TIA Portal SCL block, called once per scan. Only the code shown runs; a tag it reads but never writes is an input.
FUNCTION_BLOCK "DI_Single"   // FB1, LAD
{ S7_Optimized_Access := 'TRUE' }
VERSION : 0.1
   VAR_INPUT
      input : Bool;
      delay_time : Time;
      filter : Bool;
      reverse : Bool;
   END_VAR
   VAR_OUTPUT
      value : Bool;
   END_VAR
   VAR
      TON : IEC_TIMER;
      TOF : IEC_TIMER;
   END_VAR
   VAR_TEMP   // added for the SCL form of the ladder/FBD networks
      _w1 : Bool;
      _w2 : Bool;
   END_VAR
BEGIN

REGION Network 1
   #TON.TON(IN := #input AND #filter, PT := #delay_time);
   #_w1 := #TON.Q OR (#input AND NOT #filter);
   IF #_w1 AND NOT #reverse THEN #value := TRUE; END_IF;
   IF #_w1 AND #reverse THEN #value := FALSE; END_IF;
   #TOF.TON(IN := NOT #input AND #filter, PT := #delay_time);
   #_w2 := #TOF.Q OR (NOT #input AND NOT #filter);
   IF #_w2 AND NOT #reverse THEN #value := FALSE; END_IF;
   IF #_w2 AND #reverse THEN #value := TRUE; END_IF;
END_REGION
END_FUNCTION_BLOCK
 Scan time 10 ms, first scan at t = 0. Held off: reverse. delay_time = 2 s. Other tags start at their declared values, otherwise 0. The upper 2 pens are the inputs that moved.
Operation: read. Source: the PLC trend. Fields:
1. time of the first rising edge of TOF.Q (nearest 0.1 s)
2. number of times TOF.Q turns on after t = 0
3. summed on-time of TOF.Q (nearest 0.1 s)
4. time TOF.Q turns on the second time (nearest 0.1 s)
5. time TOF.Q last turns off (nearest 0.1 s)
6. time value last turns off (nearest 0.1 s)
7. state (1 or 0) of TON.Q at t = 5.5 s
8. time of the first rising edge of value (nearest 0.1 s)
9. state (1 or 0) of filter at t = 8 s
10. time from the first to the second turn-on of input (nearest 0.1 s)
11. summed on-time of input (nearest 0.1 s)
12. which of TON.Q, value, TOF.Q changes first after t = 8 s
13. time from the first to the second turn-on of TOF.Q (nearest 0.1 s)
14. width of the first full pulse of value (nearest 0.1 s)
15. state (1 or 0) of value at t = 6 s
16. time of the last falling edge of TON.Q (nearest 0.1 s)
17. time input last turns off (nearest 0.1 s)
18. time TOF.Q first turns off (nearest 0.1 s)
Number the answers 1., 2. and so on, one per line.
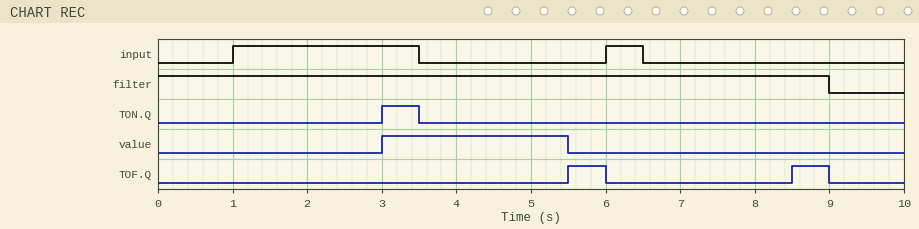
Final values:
1. 5.5 s
2. 2
3. 1.0 s
4. 8.5 s
5. 9.0 s
6. 5.5 s
7. 0
8. 3.0 s
9. 1
10. 5.0 s
11. 3.0 s
12. TOF.Q
13. 3.0 s
14. 2.5 s
15. 0
16. 3.5 s
17. 6.5 s
18. 6.0 s
